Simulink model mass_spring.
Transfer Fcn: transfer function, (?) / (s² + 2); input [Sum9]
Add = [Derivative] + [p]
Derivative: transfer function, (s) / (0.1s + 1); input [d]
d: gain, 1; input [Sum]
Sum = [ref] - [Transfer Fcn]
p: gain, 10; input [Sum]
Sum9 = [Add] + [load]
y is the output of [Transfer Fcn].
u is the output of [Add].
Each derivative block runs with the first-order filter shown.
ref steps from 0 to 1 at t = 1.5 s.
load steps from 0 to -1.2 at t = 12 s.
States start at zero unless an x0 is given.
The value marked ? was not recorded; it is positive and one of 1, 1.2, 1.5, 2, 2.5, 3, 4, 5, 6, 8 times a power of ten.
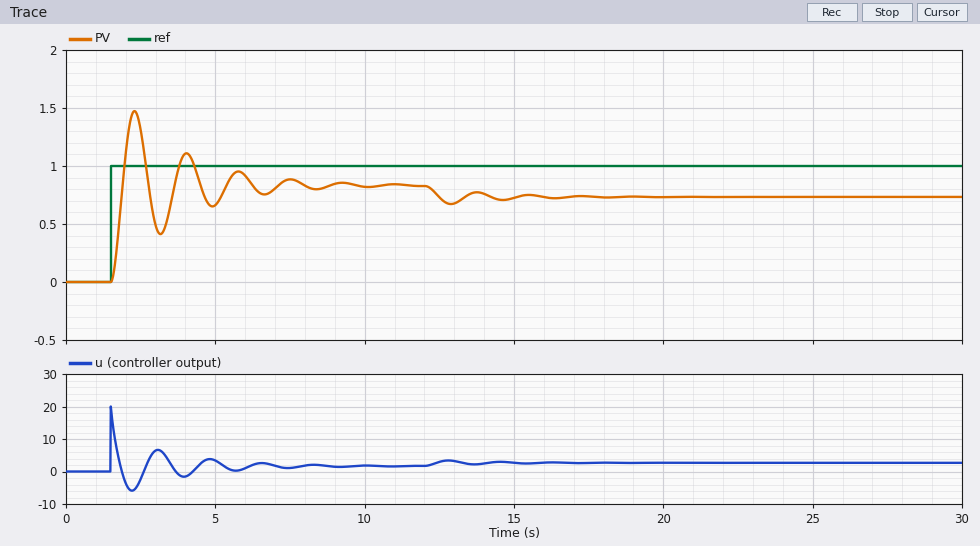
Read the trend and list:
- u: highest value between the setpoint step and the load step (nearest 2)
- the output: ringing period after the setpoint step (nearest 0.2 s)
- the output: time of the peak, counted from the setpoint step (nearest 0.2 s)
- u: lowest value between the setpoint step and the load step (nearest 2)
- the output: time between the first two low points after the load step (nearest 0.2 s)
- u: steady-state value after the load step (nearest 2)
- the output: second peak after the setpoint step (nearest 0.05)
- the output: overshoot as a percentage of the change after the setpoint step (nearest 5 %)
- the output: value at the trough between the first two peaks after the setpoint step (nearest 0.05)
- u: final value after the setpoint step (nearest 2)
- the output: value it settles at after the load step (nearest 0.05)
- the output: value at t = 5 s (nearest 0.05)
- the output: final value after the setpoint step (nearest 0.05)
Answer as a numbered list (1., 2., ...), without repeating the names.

1. 20
2. 1.8 s
3. 0.8 s
4. -6
5. 1.8 s
6. 2
7. 1.10
8. 75 %
9. 0.40
10. 2
11. 0.75
12. 0.65
13. 0.85
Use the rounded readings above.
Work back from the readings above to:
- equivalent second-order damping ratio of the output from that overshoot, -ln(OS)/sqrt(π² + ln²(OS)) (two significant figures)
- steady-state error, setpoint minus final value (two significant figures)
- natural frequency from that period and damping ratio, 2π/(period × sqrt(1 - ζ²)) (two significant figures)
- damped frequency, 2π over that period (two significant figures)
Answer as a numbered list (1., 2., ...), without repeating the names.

1. 0.091
2. 0.15
3. 3.5 rad/s
4. 3.5 rad/s
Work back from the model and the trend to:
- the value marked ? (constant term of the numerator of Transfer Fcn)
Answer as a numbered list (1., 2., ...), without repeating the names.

1. 1
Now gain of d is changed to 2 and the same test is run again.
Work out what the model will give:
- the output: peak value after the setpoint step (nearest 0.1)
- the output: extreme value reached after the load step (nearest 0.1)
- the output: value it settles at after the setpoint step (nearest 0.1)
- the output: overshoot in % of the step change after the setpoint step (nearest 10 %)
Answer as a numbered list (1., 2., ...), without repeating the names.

1. 1.4
2. 0.7
3. 0.8
4. 60 %
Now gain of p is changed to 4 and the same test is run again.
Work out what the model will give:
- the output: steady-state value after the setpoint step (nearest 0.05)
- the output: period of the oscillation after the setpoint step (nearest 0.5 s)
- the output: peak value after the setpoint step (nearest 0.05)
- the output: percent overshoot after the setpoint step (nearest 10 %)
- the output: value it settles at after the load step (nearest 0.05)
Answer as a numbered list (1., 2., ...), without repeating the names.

1. 0.65
2. 2.5 s
3. 1.15
4. 70 %
5. 0.45
